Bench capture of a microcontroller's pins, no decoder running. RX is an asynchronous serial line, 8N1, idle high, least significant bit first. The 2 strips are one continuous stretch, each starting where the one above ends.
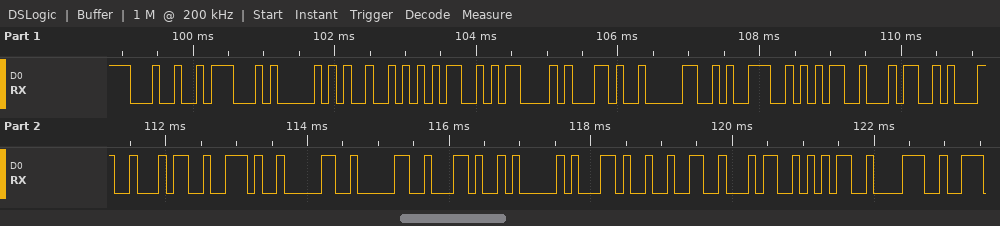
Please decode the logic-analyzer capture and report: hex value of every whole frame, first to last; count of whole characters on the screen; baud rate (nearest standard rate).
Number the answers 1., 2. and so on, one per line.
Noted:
1. 0x24 0x47 0x50 0x52 0x4D 0x43 0x2C 0x30 0x39 0x35 0x34 0x31 0x34 0x2E 0x30 0x30 0x2C 0x41 0x2C 0x32 0x34 0x35 0x38
2. 23
3. 9600 baud
